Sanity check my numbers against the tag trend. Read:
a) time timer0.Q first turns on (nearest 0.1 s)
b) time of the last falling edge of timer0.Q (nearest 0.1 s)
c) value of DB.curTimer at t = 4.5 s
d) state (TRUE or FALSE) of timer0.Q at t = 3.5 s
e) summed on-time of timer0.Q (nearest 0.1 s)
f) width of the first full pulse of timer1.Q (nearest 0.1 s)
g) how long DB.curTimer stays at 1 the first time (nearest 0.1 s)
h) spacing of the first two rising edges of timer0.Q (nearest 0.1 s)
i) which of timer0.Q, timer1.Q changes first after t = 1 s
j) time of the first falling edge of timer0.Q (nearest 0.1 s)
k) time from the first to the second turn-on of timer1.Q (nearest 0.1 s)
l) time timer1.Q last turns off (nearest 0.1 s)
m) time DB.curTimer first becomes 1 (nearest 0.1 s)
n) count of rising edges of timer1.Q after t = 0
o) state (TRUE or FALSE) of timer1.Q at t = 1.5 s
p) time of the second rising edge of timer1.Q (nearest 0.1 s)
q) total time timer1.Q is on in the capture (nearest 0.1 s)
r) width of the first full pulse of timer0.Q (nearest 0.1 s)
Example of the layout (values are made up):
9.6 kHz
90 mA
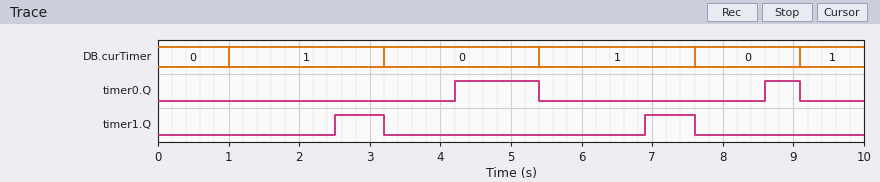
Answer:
4.2 s
9.1 s
0
FALSE
1.7 s
0.7 s
2.2 s
4.4 s
timer1.Q
5.4 s
4.4 s
7.6 s
1.0 s
2
FALSE
6.9 s
1.4 s
1.2 s
